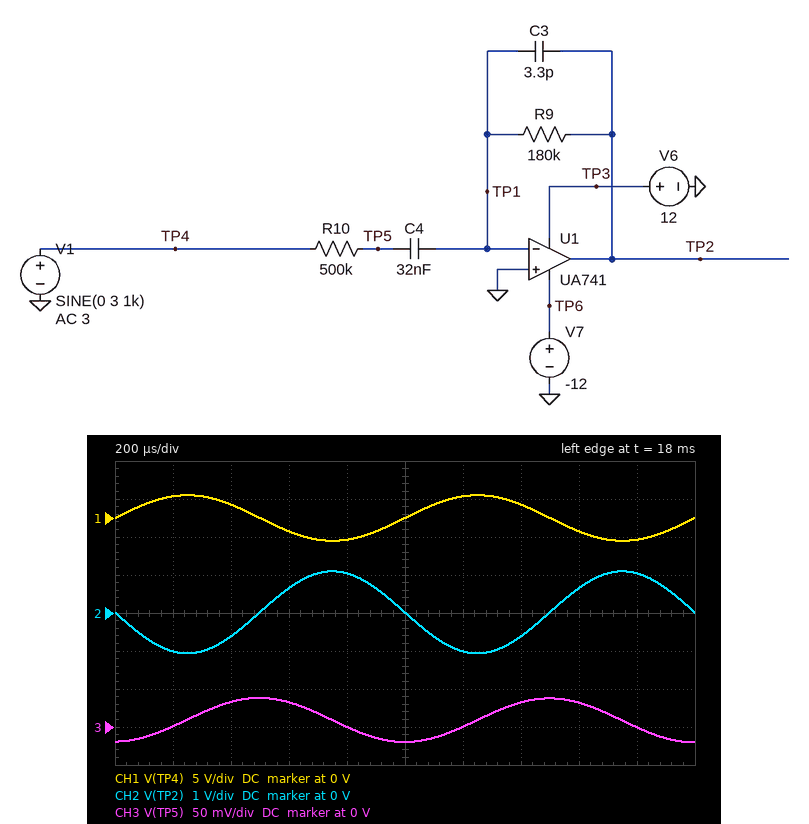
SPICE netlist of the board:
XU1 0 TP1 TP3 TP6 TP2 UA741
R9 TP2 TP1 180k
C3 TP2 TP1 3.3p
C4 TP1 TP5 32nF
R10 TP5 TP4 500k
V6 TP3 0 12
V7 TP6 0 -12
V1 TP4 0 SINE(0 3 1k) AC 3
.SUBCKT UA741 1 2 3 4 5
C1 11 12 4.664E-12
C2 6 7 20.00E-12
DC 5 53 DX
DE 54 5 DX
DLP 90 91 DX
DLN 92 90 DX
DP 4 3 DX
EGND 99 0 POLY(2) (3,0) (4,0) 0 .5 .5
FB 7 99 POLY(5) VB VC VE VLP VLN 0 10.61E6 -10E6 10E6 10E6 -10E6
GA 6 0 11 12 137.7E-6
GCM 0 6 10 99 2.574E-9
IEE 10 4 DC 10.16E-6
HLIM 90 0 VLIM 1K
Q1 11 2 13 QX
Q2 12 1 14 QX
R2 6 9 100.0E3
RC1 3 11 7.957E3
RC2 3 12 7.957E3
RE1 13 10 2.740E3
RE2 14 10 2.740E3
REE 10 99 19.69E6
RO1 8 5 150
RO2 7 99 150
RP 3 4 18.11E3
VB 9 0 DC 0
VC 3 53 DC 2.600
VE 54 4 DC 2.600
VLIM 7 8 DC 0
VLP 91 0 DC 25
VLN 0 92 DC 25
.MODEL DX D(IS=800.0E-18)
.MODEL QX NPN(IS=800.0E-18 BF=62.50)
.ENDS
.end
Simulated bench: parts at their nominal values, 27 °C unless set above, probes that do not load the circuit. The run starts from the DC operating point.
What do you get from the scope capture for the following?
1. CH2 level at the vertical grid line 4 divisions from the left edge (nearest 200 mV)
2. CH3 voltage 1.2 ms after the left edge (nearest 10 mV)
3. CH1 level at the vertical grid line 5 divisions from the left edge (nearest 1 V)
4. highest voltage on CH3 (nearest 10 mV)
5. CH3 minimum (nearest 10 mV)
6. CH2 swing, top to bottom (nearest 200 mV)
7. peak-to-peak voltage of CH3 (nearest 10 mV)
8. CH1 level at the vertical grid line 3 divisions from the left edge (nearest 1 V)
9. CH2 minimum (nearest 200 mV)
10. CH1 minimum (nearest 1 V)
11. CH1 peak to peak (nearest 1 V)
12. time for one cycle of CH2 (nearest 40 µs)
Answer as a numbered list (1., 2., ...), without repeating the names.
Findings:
1. 1.0 V
2. 0 V
3. 0 V
4. 40 mV
5. -20 mV
6. 2.2 V
7. 60 mV
8. -2 V
9. -1.0 V
10. -3 V
11. 6 V
12. 1.00 ms
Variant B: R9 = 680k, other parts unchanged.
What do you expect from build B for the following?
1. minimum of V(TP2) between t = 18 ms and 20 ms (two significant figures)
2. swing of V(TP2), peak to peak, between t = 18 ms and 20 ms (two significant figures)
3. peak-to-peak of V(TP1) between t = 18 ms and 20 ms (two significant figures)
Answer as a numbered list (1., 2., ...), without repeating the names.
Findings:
1. -4.0 V
2. 8.2 V
3. 7.5 mV
